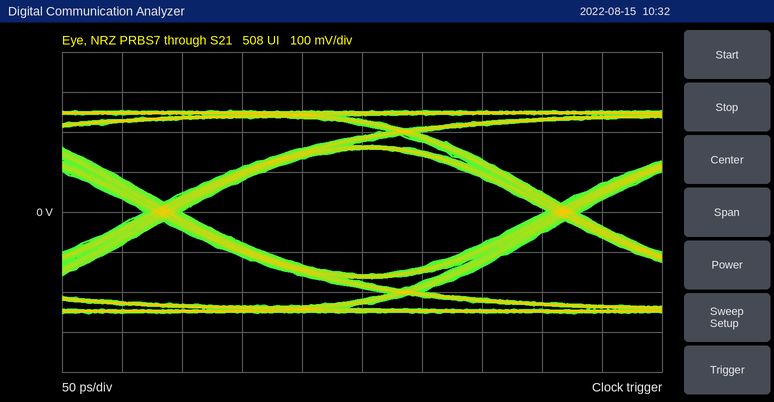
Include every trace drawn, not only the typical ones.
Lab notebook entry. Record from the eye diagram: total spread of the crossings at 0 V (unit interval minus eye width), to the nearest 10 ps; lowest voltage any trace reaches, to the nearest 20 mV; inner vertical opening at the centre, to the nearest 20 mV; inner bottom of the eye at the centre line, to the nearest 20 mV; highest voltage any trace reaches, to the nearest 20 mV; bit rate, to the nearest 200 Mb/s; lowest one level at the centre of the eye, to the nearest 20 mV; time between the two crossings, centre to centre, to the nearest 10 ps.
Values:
30 ps
-260 mV
320 mV
-160 mV
260 mV
3.0 Gb/s
160 mV
330 ps
